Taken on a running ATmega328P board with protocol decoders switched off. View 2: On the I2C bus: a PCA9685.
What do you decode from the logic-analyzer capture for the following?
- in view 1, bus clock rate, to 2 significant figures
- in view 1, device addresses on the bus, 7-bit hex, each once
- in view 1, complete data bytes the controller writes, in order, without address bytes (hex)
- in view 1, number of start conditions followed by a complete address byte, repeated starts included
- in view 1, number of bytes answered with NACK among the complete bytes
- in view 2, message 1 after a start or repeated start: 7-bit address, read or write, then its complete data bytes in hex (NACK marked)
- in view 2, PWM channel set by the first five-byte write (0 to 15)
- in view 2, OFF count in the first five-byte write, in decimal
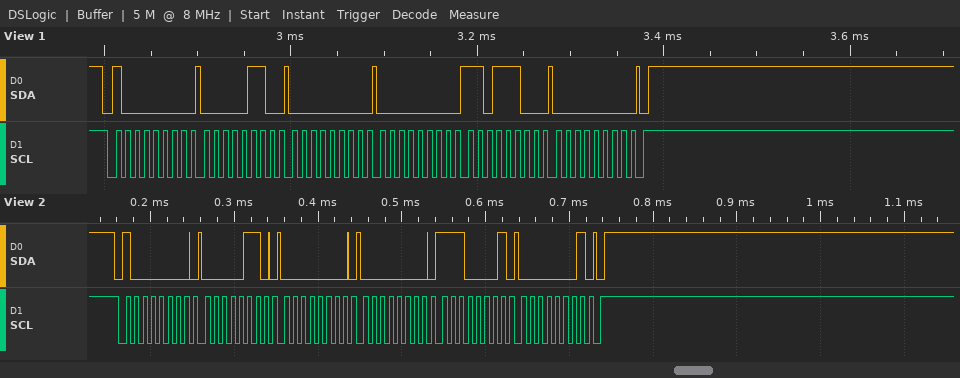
100 kHz
0x40
06 00 00 DC 00
1
0
0x40 write: 06 00 00 E1 01
0
481
